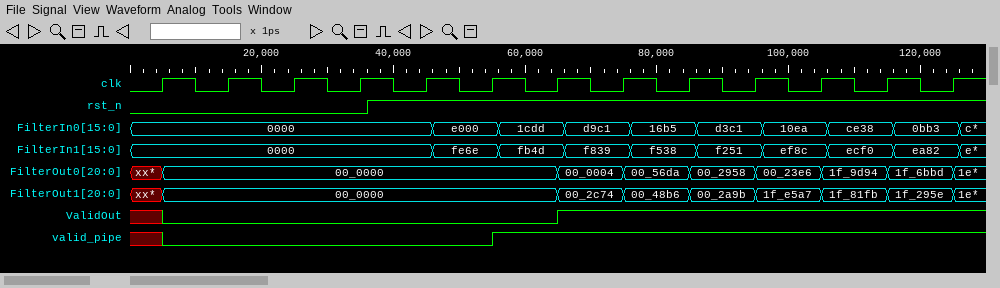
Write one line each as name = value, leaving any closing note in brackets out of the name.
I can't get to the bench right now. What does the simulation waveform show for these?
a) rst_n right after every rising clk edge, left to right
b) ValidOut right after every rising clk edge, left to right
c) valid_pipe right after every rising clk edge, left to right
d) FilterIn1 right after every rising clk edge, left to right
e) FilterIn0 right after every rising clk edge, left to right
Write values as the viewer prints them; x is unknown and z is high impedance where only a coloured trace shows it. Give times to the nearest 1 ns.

rst_n right after every rising clk edge, left to right = 0 0 0 0 1 1 1 1 1 1 1 1 1
ValidOut right after every rising clk edge, left to right = 0 0 0 0 0 0 1 1 1 1 1 1 1
valid_pipe right after every rising clk edge, left to right = 0 0 0 0 0 1 1 1 1 1 1 1 1
FilterIn1 right after every rising clk edge, left to right = 0000, 0000, 0000, 0000, 0000, fe6e, fb4d, f839, f538, f251, ef8c, ecf0, ea82
FilterIn0 right after every rising clk edge, left to right = 0000, 0000, 0000, 0000, 0000, e000, 1cdd, d9c1, 16b5, d3c1, 10ea, ce38, 0bb3
